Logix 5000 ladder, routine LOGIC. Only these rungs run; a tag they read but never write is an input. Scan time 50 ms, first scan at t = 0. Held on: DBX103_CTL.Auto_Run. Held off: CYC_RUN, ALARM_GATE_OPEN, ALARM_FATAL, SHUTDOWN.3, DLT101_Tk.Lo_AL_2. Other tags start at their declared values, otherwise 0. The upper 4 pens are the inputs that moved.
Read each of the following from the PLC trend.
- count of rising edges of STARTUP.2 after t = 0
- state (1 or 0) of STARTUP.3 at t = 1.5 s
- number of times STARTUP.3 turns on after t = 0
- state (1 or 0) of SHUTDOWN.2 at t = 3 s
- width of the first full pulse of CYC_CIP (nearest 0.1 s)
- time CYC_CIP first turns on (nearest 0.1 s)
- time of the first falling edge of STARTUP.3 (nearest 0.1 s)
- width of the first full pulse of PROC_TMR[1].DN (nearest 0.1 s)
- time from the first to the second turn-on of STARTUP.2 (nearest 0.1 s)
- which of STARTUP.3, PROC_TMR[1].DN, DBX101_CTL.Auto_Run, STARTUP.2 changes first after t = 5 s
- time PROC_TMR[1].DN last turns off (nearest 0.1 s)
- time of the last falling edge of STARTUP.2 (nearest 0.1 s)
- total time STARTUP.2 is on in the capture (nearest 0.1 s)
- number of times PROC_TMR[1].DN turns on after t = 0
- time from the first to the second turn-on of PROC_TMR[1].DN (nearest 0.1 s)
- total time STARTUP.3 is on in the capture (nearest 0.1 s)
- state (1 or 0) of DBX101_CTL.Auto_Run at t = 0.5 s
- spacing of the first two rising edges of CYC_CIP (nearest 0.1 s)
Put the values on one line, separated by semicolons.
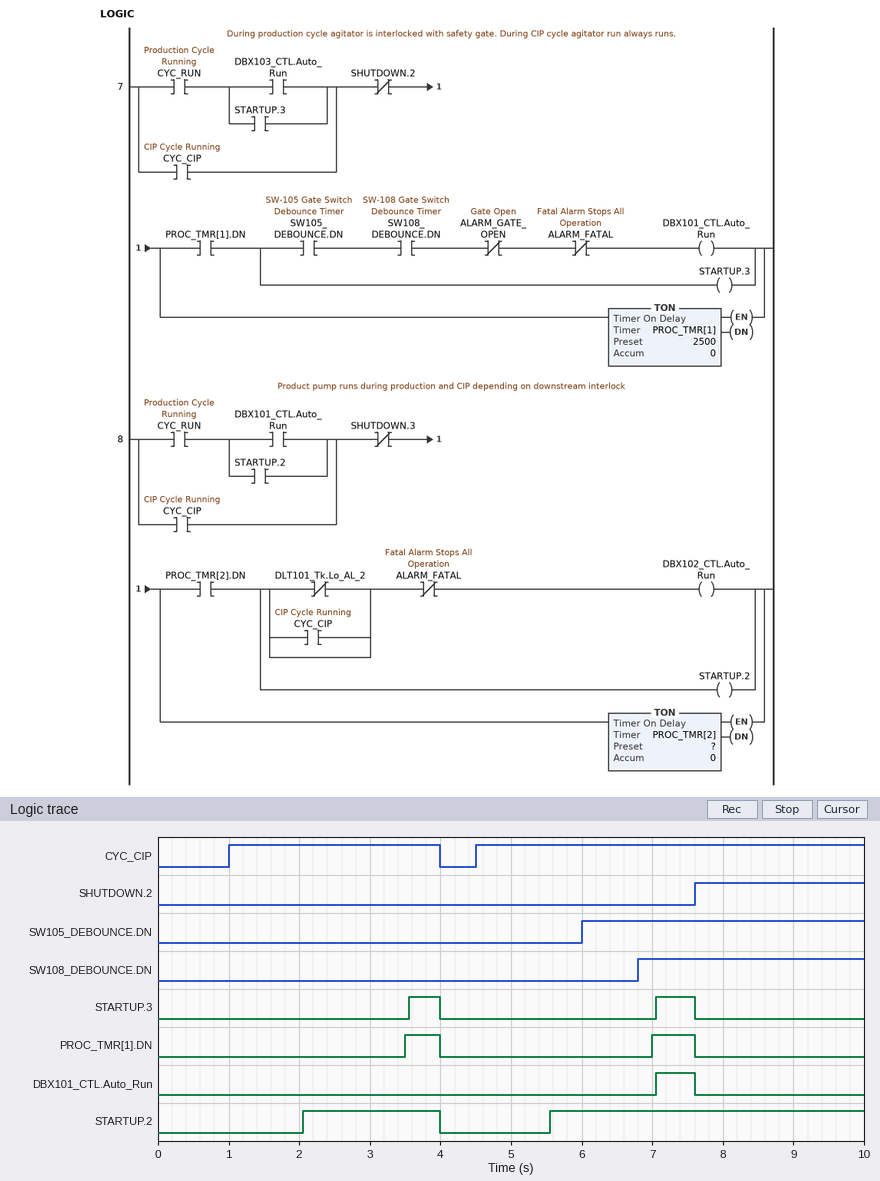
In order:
2; 0; 2; 0; 3.0 s; 1.0 s; 4.0 s; 0.5 s; 3.5 s; STARTUP.2; 7.6 s; 4.0 s; 6.4 s; 2; 3.5 s; 1.0 s; 0; 3.5 s
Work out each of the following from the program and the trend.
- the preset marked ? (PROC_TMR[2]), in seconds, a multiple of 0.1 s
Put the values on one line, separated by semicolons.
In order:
1.0 s
